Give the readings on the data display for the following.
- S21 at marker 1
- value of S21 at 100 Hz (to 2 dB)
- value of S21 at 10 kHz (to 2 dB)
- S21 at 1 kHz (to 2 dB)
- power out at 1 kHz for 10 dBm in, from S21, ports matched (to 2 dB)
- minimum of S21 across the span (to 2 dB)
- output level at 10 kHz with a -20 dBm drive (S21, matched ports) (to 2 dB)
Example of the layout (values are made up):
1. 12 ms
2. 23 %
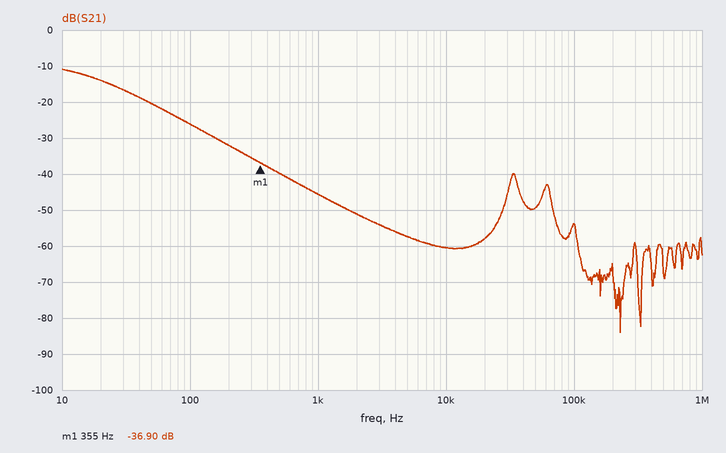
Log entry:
1. -36.90 dB
2. -26 dB
3. -60 dB
4. -46 dB
5. -36 dBm
6. -84 dB
7. -80 dBm
